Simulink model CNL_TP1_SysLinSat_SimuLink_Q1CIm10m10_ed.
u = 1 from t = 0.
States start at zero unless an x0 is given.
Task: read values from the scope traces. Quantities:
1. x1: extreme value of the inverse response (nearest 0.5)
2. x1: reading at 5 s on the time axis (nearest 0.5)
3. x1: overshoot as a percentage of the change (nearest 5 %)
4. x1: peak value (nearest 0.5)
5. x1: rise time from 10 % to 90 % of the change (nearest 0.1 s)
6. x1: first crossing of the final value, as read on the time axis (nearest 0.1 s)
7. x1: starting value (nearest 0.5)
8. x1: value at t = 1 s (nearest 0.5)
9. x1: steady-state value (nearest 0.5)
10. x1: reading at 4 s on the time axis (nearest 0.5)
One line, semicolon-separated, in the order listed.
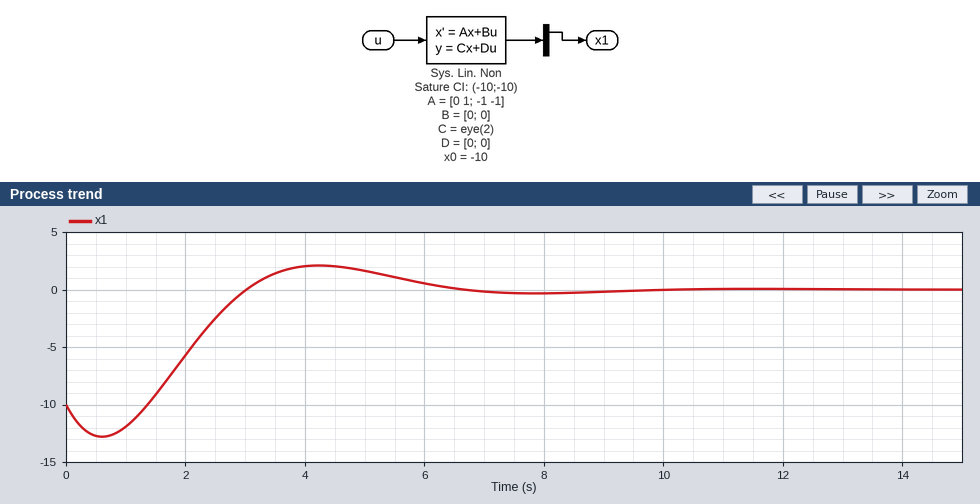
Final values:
-13.0; 1.5; 20 %; 2.0; 1.3 s; 3.0 s; -10.0; -12.0; 0.0; 2.0
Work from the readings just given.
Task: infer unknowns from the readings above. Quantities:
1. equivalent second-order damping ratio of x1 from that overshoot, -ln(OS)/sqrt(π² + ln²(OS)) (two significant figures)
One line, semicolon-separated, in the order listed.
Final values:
0.46
